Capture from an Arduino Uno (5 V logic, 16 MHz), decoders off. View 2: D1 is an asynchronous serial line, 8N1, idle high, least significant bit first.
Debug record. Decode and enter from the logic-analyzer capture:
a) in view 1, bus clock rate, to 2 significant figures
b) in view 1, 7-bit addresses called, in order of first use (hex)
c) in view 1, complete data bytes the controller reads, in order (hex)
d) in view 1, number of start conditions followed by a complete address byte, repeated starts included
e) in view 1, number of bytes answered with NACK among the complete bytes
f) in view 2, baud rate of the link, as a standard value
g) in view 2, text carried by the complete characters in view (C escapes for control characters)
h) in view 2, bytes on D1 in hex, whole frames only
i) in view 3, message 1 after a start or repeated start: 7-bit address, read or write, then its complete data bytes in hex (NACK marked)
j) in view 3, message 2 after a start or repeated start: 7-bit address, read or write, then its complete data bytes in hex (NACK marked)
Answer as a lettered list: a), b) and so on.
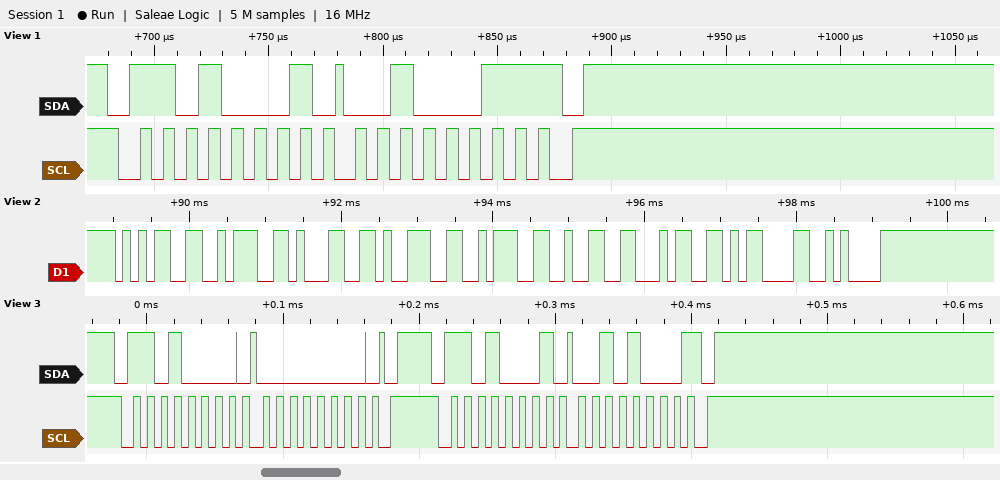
a) 100 kHz
b) 0x68
c) 23
d) 1
e) 1
f) 9600 baud
g) "5:19:24\r\n"
h) 35 3A 31 39 3A 32 34 0D 0A
i) 0x68 write: 00
j) 0x68 read: 28 NACK
